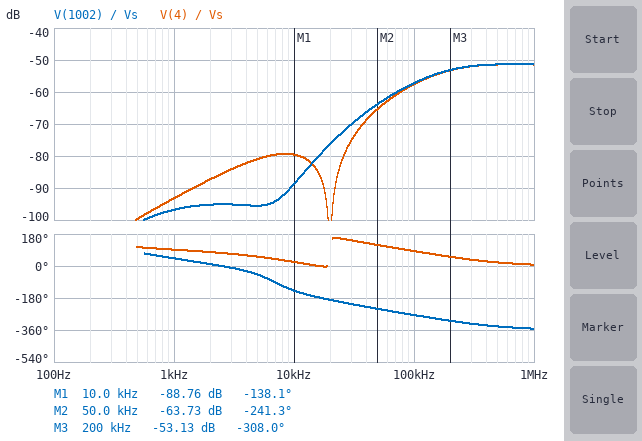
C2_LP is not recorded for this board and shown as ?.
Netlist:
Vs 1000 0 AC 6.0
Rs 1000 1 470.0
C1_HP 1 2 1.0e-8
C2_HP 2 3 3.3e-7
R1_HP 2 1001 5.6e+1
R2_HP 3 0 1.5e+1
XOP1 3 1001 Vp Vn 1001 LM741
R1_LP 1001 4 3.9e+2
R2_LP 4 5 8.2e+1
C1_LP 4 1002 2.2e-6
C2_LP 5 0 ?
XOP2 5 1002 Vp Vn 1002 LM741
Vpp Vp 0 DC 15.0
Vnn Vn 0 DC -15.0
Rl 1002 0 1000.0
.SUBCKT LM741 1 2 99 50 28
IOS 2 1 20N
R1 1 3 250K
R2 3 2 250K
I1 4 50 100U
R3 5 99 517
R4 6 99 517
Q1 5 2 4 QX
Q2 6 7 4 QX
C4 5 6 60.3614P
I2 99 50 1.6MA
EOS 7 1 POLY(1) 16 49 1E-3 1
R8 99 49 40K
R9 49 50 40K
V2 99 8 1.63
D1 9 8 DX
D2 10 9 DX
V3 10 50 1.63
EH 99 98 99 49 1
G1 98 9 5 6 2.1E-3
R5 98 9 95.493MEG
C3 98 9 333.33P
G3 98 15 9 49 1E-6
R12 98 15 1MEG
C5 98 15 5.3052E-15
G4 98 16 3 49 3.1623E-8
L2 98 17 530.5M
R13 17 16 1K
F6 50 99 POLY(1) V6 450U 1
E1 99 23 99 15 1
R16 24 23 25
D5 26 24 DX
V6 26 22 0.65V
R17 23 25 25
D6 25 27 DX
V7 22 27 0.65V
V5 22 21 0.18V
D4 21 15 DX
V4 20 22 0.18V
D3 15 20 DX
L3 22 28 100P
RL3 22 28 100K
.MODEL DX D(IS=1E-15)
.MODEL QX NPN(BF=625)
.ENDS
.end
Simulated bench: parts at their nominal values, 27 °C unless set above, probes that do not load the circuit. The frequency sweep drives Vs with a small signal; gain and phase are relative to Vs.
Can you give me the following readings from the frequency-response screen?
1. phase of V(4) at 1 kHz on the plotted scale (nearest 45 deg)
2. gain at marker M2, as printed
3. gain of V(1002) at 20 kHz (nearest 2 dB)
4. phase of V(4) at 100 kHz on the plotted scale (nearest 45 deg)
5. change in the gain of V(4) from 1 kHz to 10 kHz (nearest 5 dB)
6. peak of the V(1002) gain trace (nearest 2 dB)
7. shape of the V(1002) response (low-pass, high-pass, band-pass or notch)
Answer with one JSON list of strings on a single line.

["90 deg", "-63.73 dB", "-76 dB", "90 deg", "15 dB", "-52 dB", "high-pass"]
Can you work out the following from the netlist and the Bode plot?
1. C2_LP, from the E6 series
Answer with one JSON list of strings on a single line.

["2.2 µF"]
